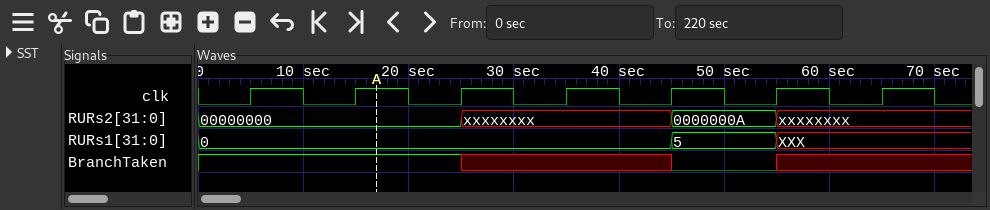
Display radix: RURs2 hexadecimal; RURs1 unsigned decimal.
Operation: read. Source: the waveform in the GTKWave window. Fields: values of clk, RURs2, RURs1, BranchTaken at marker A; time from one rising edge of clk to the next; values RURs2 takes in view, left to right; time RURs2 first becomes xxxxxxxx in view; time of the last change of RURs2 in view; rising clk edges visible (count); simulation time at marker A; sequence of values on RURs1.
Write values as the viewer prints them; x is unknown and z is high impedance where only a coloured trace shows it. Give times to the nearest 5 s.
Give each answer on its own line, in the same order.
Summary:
clk=1, RURs2=00000000, RURs1=0, BranchTaken=1
10 s
00000000, xxxxxxxx, 0000000A, xxxxxxxx
25 s
55 s
7
15 s
0, 5, XXX
